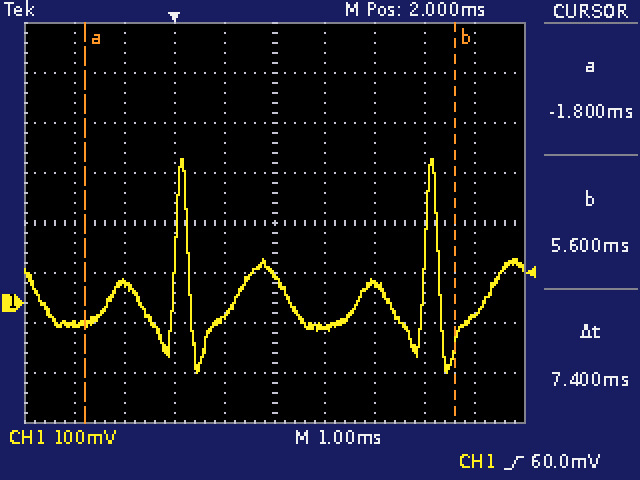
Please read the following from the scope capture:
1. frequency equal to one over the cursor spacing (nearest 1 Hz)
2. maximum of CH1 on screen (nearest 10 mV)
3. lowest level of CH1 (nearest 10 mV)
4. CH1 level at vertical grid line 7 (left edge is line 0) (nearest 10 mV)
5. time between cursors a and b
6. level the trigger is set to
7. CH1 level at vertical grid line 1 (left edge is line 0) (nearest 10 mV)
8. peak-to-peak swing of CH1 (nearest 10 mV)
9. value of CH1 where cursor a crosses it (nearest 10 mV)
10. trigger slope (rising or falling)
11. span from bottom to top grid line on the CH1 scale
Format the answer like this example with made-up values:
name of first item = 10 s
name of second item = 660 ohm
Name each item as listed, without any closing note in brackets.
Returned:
frequency equal to one over the cursor spacing = 135 Hz
maximum of CH1 on screen = 290 mV
lowest level of CH1 = -140 mV
CH1 level at vertical grid line 7 (left edge is line 0) = 40 mV
time between cursors a and b = 7.4 ms
level the trigger is set to = 60.0 mV
CH1 level at vertical grid line 1 (left edge is line 0) = -40 mV
peak-to-peak swing of CH1 = 430 mV
value of CH1 where cursor a crosses it = -40 mV
trigger slope = rising
span from bottom to top grid line on the CH1 scale = 800 mV
